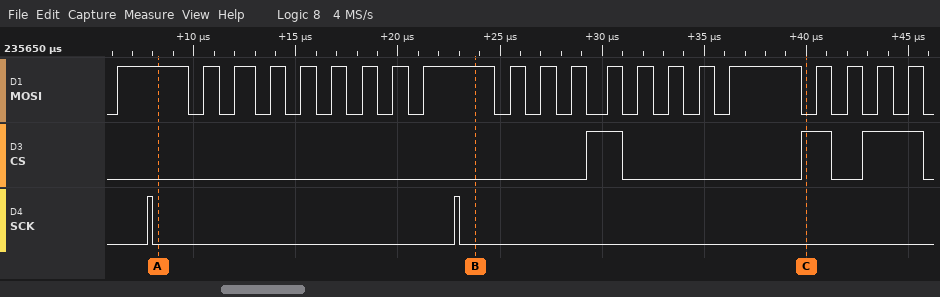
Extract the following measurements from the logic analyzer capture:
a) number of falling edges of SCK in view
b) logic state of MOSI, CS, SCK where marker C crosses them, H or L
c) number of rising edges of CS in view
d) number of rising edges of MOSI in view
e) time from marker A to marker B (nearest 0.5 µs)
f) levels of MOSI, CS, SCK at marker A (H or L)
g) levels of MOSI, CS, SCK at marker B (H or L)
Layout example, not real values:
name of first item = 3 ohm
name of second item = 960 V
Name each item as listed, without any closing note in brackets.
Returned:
number of falling edges of SCK in view = 2
logic state of MOSI, CS, SCK where marker C crosses them, H or L = MOSI=L, CS=H, SCK=L
number of rising edges of CS in view = 3
number of rising edges of MOSI in view = 21
time from marker A to marker B = 15.5 µs
levels of MOSI, CS, SCK at marker A = MOSI=H, CS=L, SCK=L
levels of MOSI, CS, SCK at marker B = MOSI=H, CS=L, SCK=L
